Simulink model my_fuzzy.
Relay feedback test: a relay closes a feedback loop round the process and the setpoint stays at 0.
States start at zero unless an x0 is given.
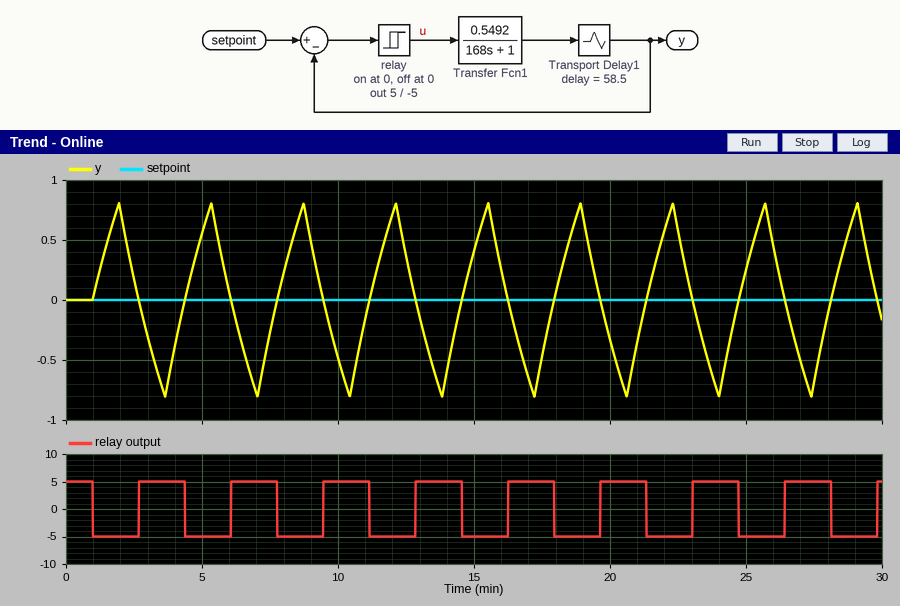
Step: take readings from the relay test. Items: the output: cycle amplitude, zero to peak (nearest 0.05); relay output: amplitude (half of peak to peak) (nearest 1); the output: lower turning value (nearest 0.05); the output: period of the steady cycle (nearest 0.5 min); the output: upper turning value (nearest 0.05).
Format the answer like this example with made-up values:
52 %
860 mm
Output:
0.80
5
-0.80
3.5 min
0.80
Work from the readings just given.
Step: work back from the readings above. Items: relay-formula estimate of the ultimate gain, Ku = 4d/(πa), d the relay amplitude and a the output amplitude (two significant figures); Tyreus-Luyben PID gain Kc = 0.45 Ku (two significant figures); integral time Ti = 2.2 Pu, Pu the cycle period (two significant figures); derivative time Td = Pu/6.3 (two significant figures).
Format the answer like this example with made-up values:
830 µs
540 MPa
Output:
8.0
3.6
7.7 min
0.56 min
